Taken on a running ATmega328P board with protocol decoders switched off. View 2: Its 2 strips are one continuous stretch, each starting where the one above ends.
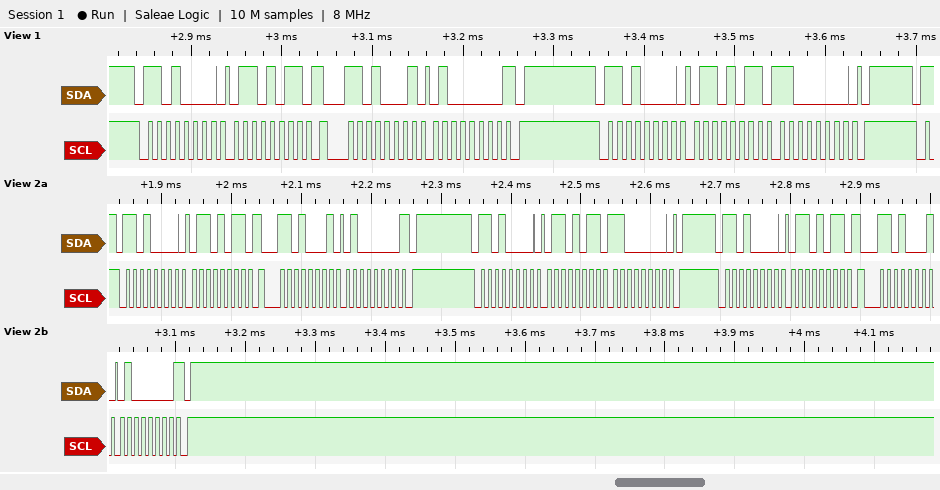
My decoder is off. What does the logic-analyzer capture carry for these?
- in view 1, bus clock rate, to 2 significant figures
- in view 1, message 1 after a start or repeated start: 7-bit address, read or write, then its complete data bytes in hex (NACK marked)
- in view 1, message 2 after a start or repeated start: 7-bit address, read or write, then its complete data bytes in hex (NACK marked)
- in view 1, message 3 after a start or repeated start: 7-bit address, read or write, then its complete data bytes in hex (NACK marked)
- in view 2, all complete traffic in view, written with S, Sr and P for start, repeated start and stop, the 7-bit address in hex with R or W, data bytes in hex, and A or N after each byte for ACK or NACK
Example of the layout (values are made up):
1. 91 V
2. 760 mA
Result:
1. 100 kHz
2. 0x68 write: 6B
3. 0x68 read: 40 NACK
4. 0x68 write: 6B C0
5. S 68W A 6B A Sr 68R A 40 N P S 68W A 6B A C0 A P S 68W A 6B A Sr 68R A 40 N P
